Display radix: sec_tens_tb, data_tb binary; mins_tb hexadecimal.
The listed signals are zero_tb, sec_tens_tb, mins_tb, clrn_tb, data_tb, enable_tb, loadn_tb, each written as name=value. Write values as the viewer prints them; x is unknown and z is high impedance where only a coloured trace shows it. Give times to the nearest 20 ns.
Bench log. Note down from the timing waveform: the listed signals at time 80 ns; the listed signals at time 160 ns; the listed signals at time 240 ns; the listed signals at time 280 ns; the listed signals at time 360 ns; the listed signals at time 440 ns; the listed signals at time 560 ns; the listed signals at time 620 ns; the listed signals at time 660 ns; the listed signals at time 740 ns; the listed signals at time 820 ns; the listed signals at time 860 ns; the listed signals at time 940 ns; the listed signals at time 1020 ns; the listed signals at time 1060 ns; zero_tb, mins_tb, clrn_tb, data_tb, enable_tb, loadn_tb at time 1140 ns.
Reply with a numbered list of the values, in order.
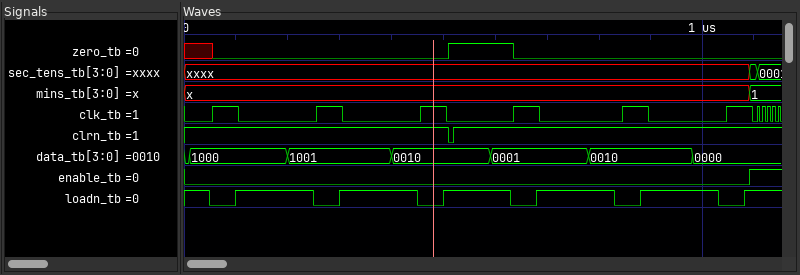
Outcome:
1. zero_tb=0, sec_tens_tb=xxxx, mins_tb=x, clrn_tb=1, data_tb=1000, enable_tb=0, loadn_tb=0
2. zero_tb=0, sec_tens_tb=xxxx, mins_tb=x, clrn_tb=1, data_tb=1000, enable_tb=0, loadn_tb=1
3. zero_tb=0, sec_tens_tb=xxxx, mins_tb=x, clrn_tb=1, data_tb=1001, enable_tb=0, loadn_tb=1
4. zero_tb=0, sec_tens_tb=xxxx, mins_tb=x, clrn_tb=1, data_tb=1001, enable_tb=0, loadn_tb=0
5. zero_tb=0, sec_tens_tb=xxxx, mins_tb=x, clrn_tb=1, data_tb=1001, enable_tb=0, loadn_tb=1
6. zero_tb=0, sec_tens_tb=xxxx, mins_tb=x, clrn_tb=1, data_tb=0010, enable_tb=0, loadn_tb=1
7. zero_tb=1, sec_tens_tb=xxxx, mins_tb=x, clrn_tb=1, data_tb=0010, enable_tb=0, loadn_tb=1
8. zero_tb=1, sec_tens_tb=xxxx, mins_tb=x, clrn_tb=1, data_tb=0001, enable_tb=0, loadn_tb=1
9. zero_tb=0, sec_tens_tb=xxxx, mins_tb=x, clrn_tb=1, data_tb=0001, enable_tb=0, loadn_tb=0
10. zero_tb=0, sec_tens_tb=xxxx, mins_tb=x, clrn_tb=1, data_tb=0001, enable_tb=0, loadn_tb=1
11. zero_tb=0, sec_tens_tb=xxxx, mins_tb=x, clrn_tb=1, data_tb=0010, enable_tb=0, loadn_tb=1
12. zero_tb=0, sec_tens_tb=xxxx, mins_tb=x, clrn_tb=1, data_tb=0010, enable_tb=0, loadn_tb=0
13. zero_tb=0, sec_tens_tb=xxxx, mins_tb=x, clrn_tb=1, data_tb=0010, enable_tb=0, loadn_tb=1
14. zero_tb=0, sec_tens_tb=xxxx, mins_tb=x, clrn_tb=1, data_tb=0000, enable_tb=0, loadn_tb=1
15. zero_tb=0, sec_tens_tb=xxxx, mins_tb=x, clrn_tb=1, data_tb=0000, enable_tb=0, loadn_tb=0
16. zero_tb=0, mins_tb=1, clrn_tb=1, data_tb=0000, enable_tb=1, loadn_tb=1
